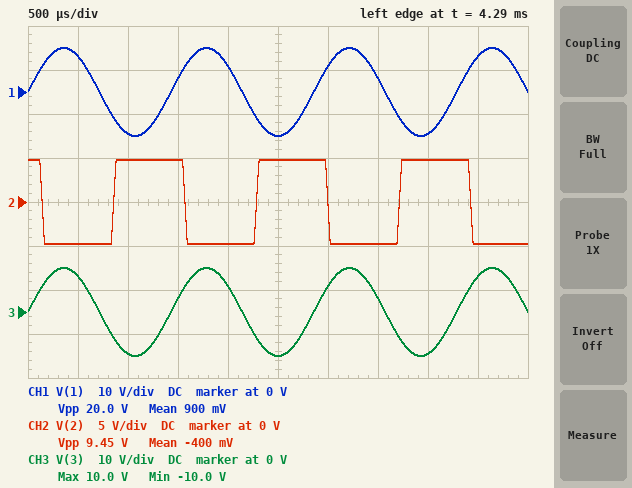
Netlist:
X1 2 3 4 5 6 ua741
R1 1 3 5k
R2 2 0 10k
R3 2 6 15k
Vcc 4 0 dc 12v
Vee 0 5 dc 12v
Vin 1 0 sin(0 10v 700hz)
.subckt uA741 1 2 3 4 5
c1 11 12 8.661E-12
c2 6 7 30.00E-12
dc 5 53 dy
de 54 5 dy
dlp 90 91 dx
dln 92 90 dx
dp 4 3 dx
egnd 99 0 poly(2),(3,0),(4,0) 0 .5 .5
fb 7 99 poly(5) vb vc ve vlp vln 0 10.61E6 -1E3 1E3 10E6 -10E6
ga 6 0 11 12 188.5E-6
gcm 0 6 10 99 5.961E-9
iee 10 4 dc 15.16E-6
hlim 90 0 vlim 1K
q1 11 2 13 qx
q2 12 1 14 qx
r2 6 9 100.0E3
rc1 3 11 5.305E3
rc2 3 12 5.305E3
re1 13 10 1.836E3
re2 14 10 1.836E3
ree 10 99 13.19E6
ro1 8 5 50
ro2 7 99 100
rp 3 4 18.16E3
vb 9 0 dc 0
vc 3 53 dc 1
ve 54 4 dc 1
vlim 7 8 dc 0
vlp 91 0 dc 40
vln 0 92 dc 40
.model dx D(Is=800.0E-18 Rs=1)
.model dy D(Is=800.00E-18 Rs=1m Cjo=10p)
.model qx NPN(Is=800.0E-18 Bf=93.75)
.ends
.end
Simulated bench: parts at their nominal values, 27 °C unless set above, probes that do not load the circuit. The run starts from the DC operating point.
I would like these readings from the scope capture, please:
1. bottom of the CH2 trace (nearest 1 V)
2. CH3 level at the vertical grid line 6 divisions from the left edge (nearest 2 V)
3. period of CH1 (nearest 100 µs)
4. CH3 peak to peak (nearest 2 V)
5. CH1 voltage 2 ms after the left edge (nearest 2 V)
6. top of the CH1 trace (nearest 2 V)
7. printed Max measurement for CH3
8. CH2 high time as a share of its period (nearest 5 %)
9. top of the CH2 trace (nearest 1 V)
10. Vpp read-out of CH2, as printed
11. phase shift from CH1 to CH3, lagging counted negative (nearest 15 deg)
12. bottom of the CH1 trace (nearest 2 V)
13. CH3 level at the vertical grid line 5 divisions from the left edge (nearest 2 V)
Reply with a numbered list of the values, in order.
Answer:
1. -5 V
2. 6 V
3. 1.4 ms
4. 20 V
5. 6 V
6. 10 V
7. 10.0 V
8. 50 %
9. 5 V
10. 9.45 V
11. 0 deg
12. -10 V
13. -10 V
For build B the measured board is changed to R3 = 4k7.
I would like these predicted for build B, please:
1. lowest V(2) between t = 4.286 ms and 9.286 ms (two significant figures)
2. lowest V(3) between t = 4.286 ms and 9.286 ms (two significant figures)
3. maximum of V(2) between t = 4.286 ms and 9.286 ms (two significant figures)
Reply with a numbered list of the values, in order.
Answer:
1. -8.0 V
2. -10 V
3. 8.0 V
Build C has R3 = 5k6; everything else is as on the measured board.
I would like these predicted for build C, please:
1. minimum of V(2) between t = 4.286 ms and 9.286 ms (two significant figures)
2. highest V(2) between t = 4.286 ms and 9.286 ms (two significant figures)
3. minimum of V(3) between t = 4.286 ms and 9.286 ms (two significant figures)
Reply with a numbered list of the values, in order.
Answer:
1. -7.6 V
2. 7.6 V
3. -10 V
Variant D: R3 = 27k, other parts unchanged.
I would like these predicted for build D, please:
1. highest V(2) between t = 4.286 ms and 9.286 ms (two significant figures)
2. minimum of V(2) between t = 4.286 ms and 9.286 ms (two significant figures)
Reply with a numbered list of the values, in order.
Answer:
1. 3.2 V
2. -3.2 V
